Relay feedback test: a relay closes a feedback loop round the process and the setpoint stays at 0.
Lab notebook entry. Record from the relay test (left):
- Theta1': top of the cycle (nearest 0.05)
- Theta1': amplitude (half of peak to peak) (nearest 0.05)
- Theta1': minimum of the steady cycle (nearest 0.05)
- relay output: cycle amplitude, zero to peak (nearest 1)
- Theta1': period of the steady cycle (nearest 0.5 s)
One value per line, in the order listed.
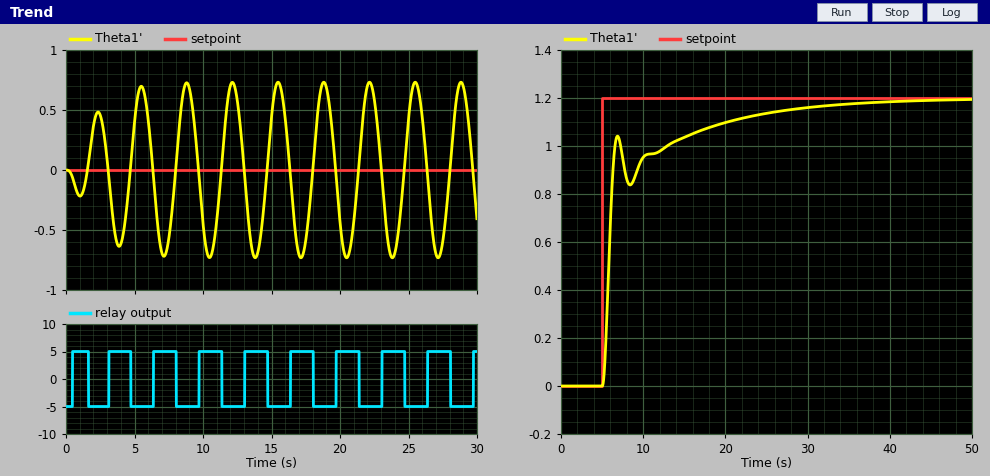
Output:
0.75
0.75
-0.75
5
3.5 s
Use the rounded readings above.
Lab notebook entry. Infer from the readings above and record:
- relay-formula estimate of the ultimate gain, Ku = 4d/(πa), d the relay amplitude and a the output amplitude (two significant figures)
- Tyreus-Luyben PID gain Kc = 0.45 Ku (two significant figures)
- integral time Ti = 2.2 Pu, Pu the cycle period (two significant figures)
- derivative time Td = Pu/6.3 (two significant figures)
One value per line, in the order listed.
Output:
8.5
3.8
7.7 s
0.56 s
